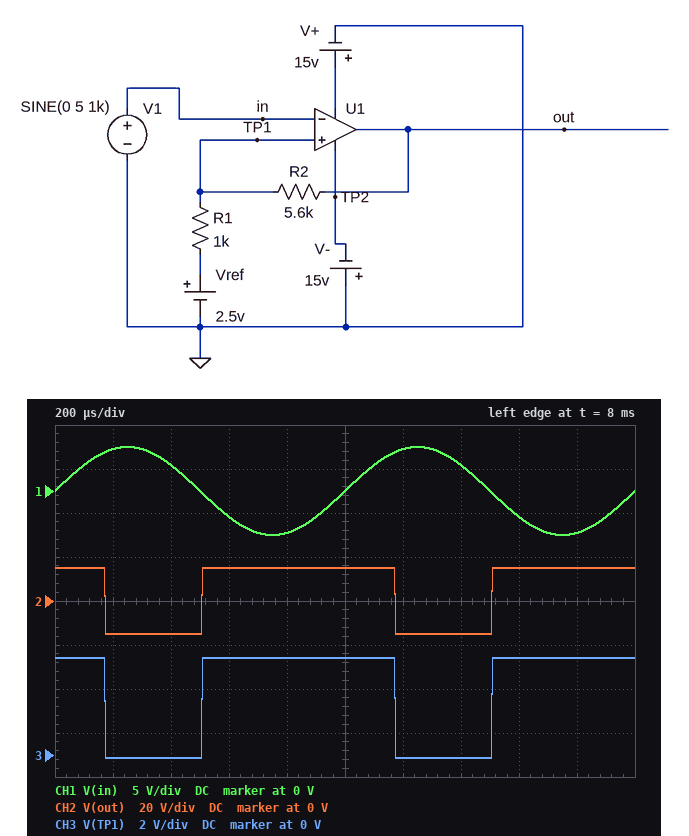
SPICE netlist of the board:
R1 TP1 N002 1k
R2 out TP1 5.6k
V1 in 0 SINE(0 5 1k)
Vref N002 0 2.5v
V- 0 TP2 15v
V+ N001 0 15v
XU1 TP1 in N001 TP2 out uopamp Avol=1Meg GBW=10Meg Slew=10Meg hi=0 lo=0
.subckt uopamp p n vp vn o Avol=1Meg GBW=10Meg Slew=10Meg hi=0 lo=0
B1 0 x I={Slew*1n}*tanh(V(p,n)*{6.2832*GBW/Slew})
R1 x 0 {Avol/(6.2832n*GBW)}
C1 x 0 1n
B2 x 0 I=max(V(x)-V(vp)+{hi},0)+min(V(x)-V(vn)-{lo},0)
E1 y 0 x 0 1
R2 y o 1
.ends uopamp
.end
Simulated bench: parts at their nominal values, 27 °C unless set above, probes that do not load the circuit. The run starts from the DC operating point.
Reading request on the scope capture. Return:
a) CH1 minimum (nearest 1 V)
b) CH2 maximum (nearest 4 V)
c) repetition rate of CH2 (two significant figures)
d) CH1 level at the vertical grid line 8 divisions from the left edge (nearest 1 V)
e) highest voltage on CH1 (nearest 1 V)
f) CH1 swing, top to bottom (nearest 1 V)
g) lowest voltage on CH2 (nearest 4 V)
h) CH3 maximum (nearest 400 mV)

-5 V
16 V
1.0 kHz
-3 V
5 V
10 V
-16 V
4.4 V
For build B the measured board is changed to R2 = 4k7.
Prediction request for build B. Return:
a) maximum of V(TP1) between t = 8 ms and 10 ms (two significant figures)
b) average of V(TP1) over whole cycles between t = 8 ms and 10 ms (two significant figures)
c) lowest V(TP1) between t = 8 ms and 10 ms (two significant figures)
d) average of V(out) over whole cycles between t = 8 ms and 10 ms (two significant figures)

4.7 V
3.0 V
-570 mV
5.3 V
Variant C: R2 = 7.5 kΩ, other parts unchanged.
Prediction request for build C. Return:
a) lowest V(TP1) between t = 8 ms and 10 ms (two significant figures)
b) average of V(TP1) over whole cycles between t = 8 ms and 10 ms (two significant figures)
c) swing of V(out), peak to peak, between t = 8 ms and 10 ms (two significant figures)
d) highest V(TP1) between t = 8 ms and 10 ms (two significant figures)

440 mV
2.8 V
30 V
4.0 V
